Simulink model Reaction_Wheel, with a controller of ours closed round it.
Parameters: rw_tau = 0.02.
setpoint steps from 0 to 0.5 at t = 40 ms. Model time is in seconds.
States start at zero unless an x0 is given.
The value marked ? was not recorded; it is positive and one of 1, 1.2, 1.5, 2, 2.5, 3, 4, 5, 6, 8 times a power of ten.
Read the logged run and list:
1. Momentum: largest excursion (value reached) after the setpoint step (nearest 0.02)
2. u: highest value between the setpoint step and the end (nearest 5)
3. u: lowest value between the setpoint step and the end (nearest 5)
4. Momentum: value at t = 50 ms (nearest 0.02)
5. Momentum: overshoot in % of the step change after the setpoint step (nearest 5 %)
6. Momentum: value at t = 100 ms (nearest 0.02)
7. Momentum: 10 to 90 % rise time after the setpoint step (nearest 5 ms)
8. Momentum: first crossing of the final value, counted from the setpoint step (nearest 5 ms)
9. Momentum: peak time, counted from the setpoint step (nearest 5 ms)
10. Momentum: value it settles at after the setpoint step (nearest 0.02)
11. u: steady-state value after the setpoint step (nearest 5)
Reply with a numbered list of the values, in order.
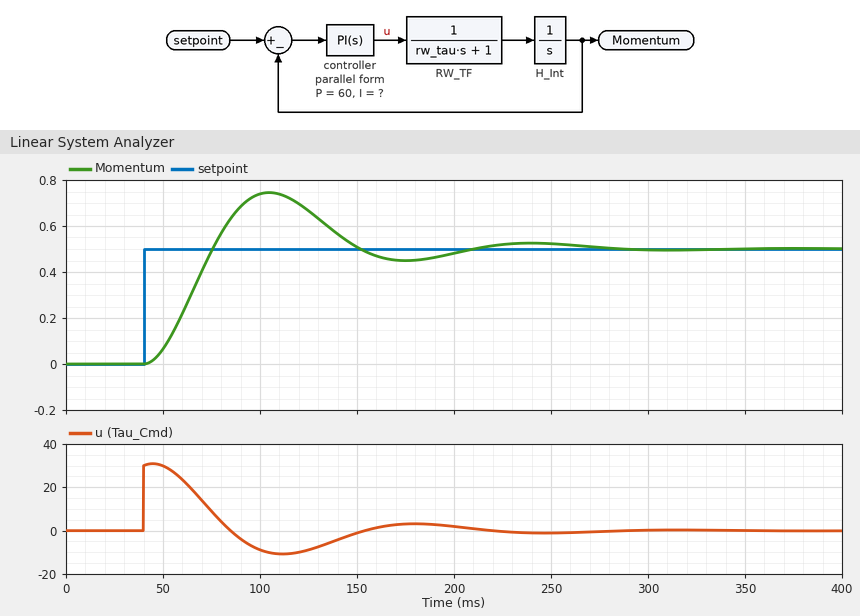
1. 0.74
2. 30
3. -10
4. 0.06
5. 50 %
6. 0.74
7. 25 ms
8. 35 ms
9. 65 ms
10. 0.50
11. 0
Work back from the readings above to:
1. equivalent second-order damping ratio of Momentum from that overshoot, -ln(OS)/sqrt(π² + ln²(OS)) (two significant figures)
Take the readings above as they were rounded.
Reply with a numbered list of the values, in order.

1. 0.22
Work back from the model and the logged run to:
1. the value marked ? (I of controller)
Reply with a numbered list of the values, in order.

1. 800
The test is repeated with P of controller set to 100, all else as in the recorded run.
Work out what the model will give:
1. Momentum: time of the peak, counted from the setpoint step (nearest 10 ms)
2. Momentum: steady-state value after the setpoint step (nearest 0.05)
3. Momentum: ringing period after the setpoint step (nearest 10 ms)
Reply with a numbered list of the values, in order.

1. 50 ms
2. 0.50
3. 100 ms
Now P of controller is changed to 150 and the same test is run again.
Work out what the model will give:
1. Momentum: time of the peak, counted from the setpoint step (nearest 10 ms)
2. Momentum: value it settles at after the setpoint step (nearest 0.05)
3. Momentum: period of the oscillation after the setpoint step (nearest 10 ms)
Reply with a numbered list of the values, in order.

1. 40 ms
2. 0.50
3. 80 ms
